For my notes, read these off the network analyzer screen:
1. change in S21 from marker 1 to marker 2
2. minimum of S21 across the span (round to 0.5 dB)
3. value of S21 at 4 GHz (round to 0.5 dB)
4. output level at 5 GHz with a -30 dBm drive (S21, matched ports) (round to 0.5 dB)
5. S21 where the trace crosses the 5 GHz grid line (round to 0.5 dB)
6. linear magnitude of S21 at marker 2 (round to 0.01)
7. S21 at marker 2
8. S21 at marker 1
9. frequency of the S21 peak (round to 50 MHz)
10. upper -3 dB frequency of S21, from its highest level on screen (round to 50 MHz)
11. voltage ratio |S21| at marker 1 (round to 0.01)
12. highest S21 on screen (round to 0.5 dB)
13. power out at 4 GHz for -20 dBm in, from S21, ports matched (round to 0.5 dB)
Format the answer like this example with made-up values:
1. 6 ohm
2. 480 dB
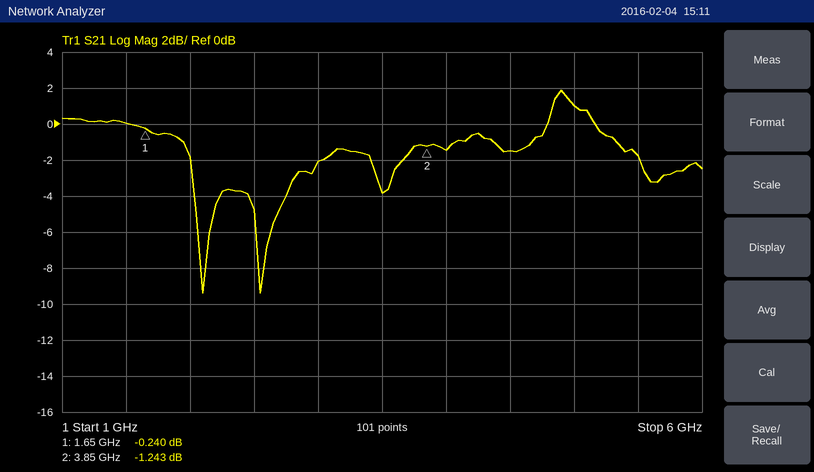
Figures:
1. -1.003 dB
2. -9.5 dB
3. -1.5 dB
4. -29.0 dBm
5. 1.0 dB
6. 0.87
7. -1.243 dB
8. -0.240 dB
9. 4.90 GHz
10. 5.35 GHz
11. 0.97
12. 2.0 dB
13. -21.5 dBm
